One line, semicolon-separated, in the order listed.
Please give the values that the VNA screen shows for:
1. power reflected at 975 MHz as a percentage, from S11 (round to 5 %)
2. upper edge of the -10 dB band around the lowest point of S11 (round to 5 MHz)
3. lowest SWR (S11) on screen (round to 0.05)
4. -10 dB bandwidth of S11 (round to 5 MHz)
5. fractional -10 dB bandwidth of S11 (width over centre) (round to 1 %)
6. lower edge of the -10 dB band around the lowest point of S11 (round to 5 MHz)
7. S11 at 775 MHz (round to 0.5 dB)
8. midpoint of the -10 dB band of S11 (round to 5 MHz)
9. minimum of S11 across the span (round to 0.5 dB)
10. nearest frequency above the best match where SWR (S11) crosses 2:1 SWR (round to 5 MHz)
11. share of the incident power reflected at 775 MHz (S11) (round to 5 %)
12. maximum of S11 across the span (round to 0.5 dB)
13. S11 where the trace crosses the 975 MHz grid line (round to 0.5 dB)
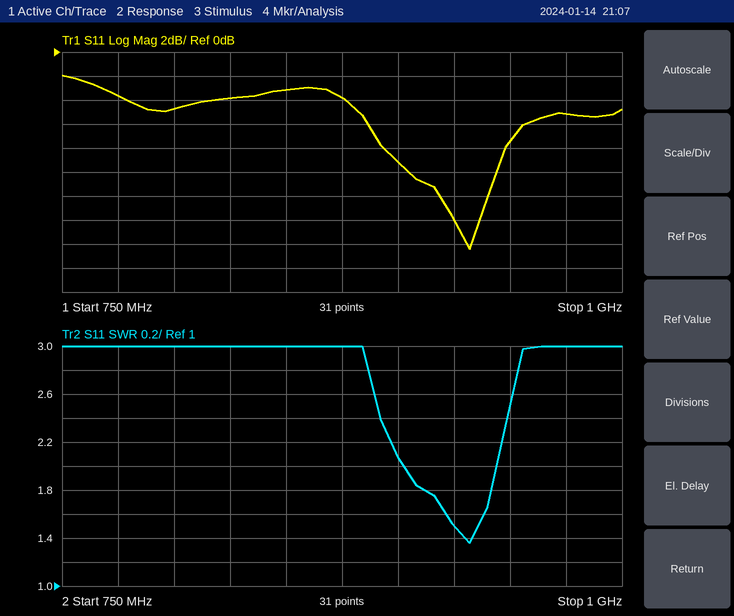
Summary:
30 %; 945 MHz; 1.35; 40 MHz; 4 %; 905 MHz; -3.5 dB; 925 MHz; -16.5 dB; 945 MHz; 45 %; -2.0 dB; -5.0 dB
